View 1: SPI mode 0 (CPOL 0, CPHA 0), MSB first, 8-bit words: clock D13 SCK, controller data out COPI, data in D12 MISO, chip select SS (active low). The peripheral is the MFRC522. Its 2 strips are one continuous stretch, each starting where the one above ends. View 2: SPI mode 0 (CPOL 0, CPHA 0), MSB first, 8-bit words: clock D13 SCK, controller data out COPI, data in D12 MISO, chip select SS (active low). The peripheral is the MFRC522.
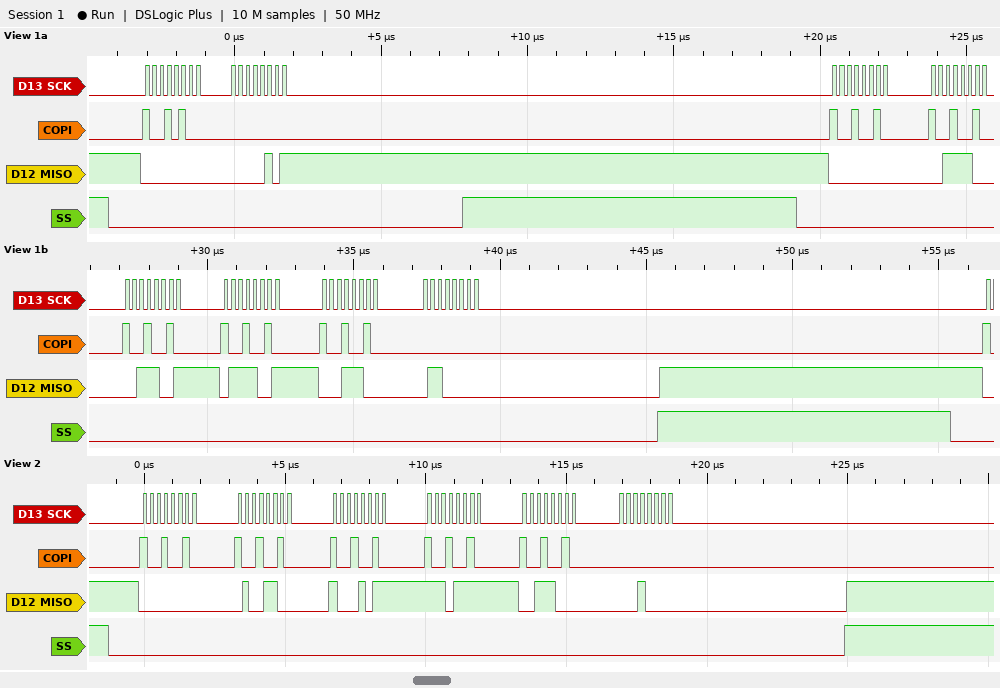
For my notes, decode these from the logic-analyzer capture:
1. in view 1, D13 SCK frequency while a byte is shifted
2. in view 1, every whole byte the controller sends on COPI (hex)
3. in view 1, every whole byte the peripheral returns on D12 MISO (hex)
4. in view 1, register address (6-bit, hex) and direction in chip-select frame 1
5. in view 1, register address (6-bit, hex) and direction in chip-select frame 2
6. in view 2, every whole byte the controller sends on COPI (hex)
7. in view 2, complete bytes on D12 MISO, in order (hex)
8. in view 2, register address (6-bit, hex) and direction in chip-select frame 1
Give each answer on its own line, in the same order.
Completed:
4 MHz
94 00 92 92 92 92 92 00
00 05 00 3C 39 79 1C 60
0x0A read
0x09 read
92 92 92 92 92 00
00 4C 8B EF 38 10
0x09 read
